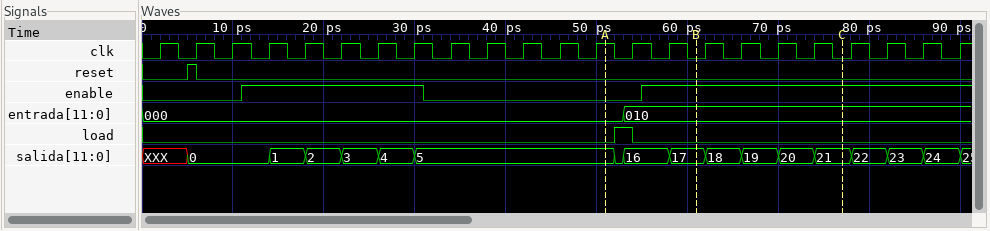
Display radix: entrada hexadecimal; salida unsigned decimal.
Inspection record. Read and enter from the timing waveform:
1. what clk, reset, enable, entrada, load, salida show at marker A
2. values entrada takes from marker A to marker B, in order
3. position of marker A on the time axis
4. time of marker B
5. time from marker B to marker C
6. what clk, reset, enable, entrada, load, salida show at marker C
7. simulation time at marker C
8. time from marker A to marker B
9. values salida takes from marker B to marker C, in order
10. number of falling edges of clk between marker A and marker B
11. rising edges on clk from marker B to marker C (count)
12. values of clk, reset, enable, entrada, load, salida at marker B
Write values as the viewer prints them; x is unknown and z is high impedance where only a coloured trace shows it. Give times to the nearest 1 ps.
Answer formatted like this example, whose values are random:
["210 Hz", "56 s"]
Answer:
["clk=1, reset=0, enable=0, entrada=000, load=0, salida=5", "000, 010", "51 ps", "61 ps", "16 ps", "clk=0, reset=0, enable=1, entrada=010, load=0, salida=21", "77 ps", "10 ps", "17, 18, 19, 20, 21", "3", "4", "clk=0, reset=0, enable=1, entrada=010, load=0, salida=17"]
